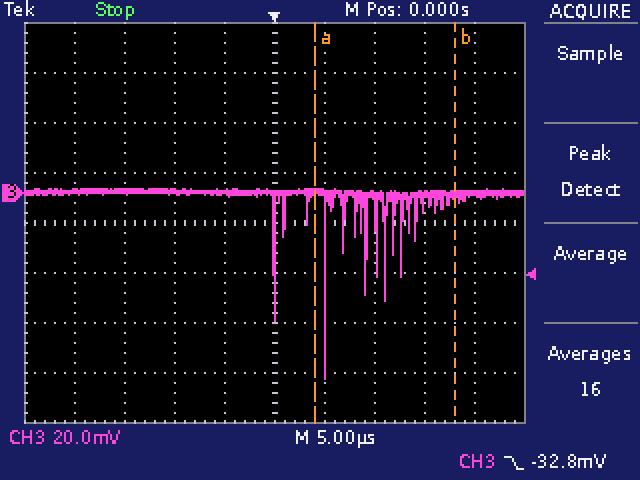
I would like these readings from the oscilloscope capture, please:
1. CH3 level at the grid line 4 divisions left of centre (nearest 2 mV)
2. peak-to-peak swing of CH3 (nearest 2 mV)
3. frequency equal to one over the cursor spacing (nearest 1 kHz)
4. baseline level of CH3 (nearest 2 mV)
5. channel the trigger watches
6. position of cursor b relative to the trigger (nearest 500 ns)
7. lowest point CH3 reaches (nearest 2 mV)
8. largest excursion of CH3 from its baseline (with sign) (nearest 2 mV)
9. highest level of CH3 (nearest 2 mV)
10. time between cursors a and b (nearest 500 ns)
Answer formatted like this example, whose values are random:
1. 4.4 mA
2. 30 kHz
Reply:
1. 0 mV
2. 76 mV
3. 71 kHz
4. 0 mV
5. CH3
6. +18.0 µs
7. -74 mV
8. -74 mV
9. 2 mV
10. 14.0 µs
